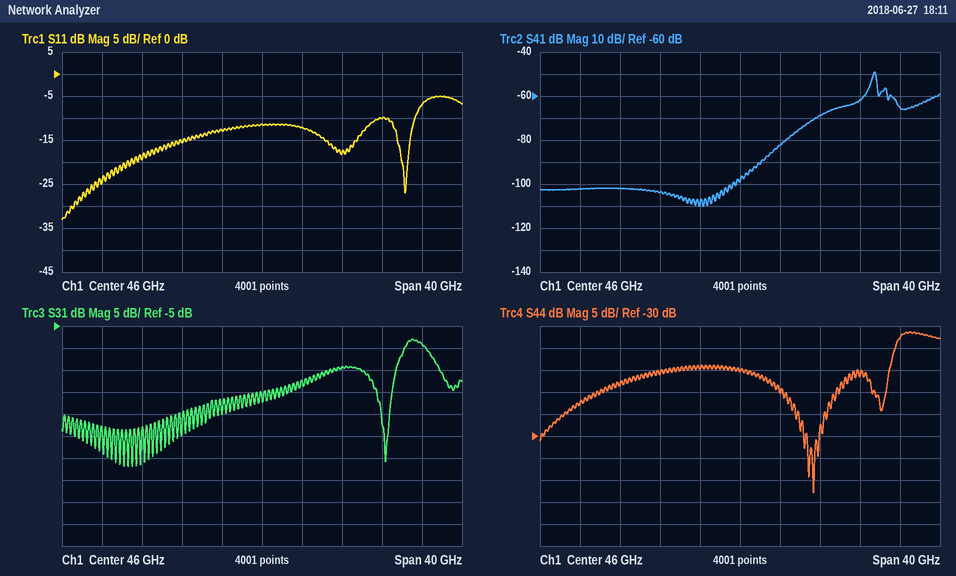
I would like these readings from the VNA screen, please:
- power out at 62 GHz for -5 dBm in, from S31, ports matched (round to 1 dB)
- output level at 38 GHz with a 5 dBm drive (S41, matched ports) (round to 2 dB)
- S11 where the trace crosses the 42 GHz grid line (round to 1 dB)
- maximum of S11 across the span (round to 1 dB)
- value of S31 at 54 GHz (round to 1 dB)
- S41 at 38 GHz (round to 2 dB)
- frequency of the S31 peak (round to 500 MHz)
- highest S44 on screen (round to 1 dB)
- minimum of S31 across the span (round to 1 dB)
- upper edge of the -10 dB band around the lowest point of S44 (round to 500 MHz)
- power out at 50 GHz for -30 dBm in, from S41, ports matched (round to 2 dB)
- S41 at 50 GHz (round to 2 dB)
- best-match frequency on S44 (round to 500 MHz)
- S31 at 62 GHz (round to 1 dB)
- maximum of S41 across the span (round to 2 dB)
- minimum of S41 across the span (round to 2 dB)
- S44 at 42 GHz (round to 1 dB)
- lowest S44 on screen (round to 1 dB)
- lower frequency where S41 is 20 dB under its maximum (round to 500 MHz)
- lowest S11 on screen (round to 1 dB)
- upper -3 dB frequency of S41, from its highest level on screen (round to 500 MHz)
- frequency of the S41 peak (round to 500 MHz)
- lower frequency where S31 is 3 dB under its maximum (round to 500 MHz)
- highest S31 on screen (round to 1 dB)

-14 dBm
-98 dBm
-13 dB
-5 dB
-14 dB
-104 dB
61.0 GHz
-6 dB
-37 dB
61.5 GHz
-112 dBm
-82 dB
53.5 GHz
-9 dB
-50 dB
-110 dB
-15 dB
-43 dB
54.0 GHz
-33 dB
59.5 GHz
59.5 GHz
60.0 GHz
-8 dB
